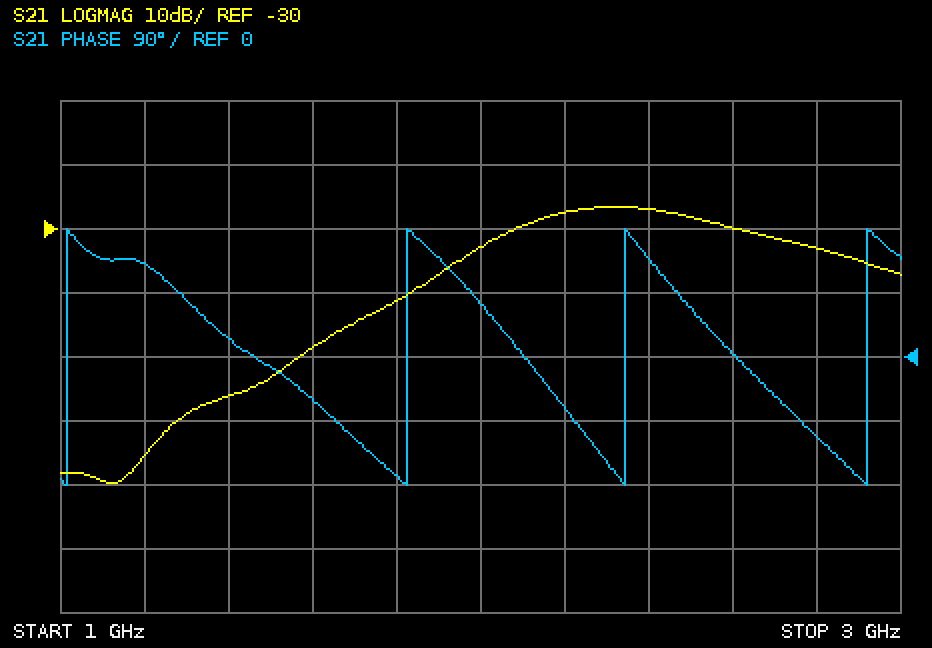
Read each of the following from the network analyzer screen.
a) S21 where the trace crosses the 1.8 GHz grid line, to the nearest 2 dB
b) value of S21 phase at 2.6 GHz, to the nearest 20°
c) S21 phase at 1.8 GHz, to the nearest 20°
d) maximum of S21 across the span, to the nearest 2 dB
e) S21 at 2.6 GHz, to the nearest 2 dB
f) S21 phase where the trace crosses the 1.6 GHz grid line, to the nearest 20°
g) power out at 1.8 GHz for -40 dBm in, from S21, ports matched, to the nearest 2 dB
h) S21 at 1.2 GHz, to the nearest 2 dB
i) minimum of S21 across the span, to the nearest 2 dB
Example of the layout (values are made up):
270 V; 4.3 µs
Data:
-42 dB; 0°; -160°; -26 dB; -30 dB; -60°; -82 dBm; -66 dB; -70 dB
